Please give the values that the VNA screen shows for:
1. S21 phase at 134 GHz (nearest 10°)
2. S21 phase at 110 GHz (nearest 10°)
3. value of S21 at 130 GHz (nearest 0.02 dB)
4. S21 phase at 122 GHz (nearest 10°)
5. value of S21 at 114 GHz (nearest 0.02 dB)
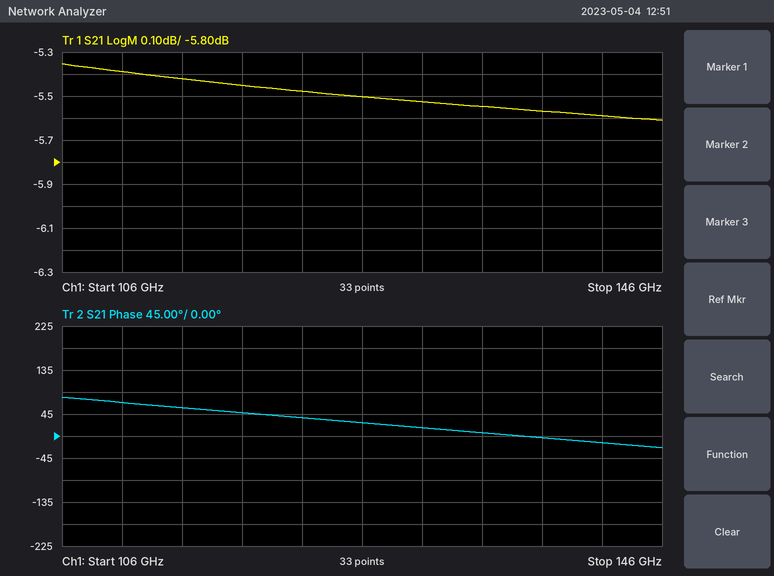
10°
70°
-5.52 dB
40°
-5.42 dB
